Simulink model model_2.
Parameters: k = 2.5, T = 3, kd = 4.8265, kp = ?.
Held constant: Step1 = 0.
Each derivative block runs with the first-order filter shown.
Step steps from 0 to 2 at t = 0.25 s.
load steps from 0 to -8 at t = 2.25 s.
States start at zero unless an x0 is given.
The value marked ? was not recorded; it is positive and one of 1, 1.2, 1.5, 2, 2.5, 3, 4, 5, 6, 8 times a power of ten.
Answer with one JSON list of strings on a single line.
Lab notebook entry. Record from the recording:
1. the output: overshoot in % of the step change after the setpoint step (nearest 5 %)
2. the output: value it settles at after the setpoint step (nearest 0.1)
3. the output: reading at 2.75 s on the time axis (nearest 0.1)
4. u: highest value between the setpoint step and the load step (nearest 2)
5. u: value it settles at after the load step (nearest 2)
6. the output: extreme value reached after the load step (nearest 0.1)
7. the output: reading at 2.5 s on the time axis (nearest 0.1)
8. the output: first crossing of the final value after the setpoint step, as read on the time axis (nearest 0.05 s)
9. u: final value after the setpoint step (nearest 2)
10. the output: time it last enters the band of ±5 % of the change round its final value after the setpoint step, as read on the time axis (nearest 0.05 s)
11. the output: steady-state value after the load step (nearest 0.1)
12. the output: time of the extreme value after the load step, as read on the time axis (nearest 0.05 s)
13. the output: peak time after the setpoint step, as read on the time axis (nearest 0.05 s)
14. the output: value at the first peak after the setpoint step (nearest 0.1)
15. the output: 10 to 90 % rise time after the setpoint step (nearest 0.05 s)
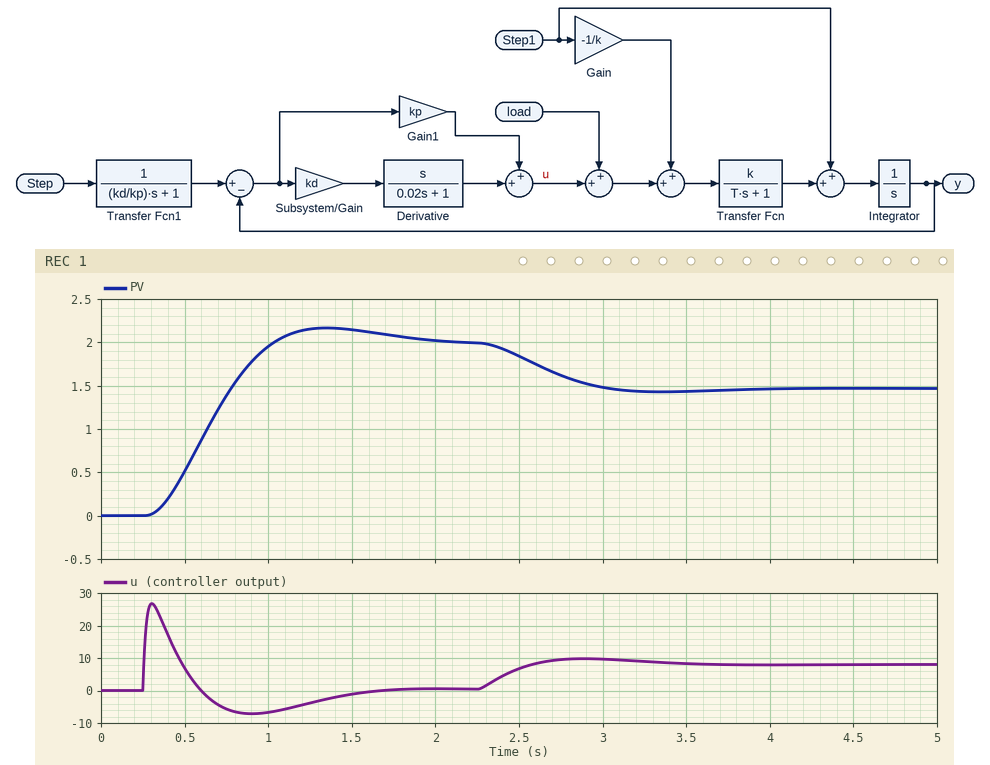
["10 %", "2.0", "1.6", "26", "8", "1.4", "1.8", "1.05 s", "0", "1.65 s", "1.5", "3.35 s", "1.35 s", "2.2", "0.50 s"]
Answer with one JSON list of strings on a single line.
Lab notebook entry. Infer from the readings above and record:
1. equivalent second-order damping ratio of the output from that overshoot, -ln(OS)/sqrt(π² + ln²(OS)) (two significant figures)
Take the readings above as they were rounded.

["0.59"]
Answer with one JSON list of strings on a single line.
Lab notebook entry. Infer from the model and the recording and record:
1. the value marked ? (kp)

["15"]
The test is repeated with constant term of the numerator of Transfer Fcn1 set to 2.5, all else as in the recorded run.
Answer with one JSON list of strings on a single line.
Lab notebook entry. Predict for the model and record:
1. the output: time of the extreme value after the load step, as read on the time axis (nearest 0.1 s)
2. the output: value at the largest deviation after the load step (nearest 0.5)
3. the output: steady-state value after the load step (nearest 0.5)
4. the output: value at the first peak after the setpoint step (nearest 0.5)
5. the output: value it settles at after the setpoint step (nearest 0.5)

["3.3 s", "4.5", "4.5", "5.5", "5.0"]
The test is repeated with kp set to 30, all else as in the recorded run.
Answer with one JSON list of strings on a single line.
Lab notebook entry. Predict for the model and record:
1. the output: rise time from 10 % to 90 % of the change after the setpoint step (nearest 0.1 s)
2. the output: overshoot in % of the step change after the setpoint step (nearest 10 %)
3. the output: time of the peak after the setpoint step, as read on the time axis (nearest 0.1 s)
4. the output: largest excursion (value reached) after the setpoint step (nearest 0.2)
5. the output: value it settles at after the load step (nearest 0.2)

["0.3 s", "20 %", "0.9 s", "2.4", "1.8"]
